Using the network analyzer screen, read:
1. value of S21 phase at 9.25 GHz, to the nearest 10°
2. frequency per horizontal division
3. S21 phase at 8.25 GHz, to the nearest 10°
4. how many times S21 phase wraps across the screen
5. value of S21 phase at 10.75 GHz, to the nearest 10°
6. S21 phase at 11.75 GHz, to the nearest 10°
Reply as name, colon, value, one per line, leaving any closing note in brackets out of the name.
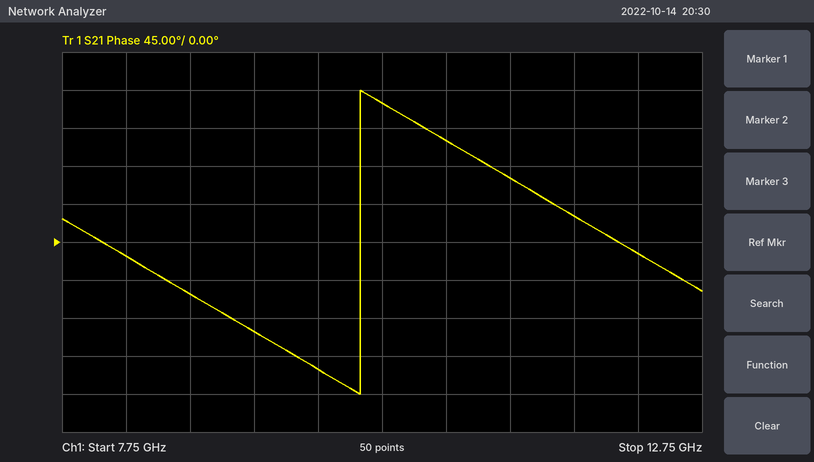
value of S21 phase at 9.25 GHz, to the nearest 10°: -110°
frequency per horizontal division: 500 MHz
S21 phase at 8.25 GHz, to the nearest 10°: -20°
how many times S21 phase wraps across the screen: 1
value of S21 phase at 10.75 GHz, to the nearest 10°: 120°
S21 phase at 11.75 GHz, to the nearest 10°: 30°
